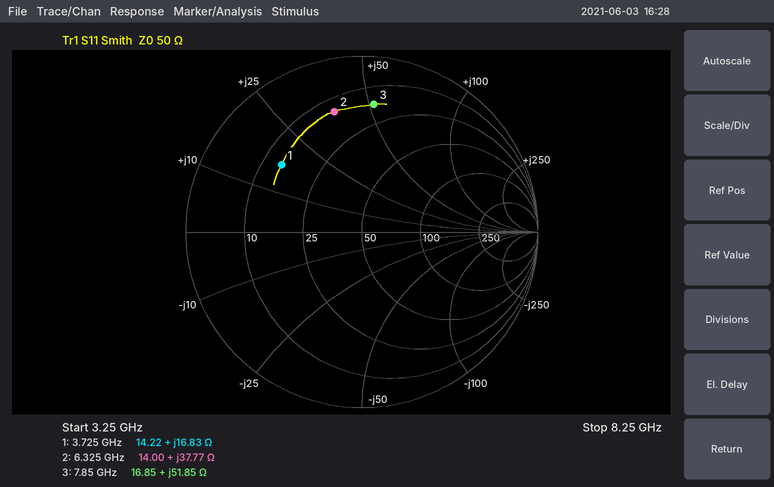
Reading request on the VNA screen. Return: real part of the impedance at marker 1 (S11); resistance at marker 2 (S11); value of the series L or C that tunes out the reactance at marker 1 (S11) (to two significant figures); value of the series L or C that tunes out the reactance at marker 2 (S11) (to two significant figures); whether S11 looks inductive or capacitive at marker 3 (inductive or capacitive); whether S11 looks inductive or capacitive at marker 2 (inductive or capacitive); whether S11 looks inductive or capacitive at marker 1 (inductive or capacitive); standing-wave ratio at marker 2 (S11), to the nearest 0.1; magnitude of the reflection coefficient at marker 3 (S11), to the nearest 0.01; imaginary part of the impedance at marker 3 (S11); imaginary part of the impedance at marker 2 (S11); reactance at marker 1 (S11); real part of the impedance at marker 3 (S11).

14.22 Ω
14.00 Ω
2.5 pF
670 fF
inductive
inductive
inductive
5.7
0.73
+51.85 Ω
+37.77 Ω
+16.83 Ω
16.85 Ω
